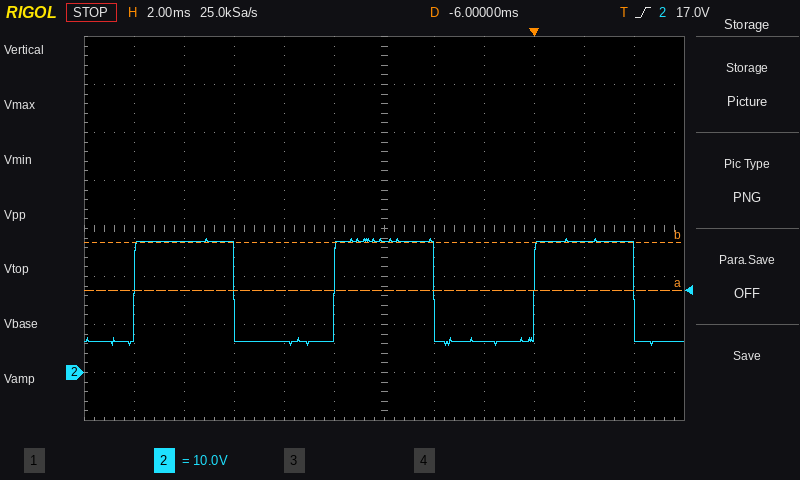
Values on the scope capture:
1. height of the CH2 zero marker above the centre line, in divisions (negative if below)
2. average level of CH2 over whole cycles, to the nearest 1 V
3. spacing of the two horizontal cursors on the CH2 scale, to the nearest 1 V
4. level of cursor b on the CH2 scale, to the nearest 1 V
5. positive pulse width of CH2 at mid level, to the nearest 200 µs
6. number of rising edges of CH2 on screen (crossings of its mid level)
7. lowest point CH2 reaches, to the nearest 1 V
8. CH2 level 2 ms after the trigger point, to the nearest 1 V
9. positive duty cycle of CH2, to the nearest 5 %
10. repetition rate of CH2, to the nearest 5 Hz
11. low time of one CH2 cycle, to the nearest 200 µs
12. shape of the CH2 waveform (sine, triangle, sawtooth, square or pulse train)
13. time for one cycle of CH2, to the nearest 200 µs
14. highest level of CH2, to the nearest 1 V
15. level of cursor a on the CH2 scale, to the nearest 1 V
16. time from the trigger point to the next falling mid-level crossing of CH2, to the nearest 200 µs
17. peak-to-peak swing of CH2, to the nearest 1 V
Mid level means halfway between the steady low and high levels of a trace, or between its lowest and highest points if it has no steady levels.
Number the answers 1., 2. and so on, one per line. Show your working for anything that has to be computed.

1. -3.0 div
2. 6 V + 0.5 × (28 V − (6 V)) ≈ 17 V
3. 10 V
4. 27 V
5. 4.0 ms
6. 3
7. 6 V
8. 27 V
9. 4.0 ms / 8.0 ms ≈ 50 %
10. 1 / 8.0 ms ≈ 125 Hz
11. 4.0 ms
12. square
13. 8.0 ms
14. 28 V
15. 17 V
16. 4.0 ms
17. 28 V − (6 V) = 22 V
